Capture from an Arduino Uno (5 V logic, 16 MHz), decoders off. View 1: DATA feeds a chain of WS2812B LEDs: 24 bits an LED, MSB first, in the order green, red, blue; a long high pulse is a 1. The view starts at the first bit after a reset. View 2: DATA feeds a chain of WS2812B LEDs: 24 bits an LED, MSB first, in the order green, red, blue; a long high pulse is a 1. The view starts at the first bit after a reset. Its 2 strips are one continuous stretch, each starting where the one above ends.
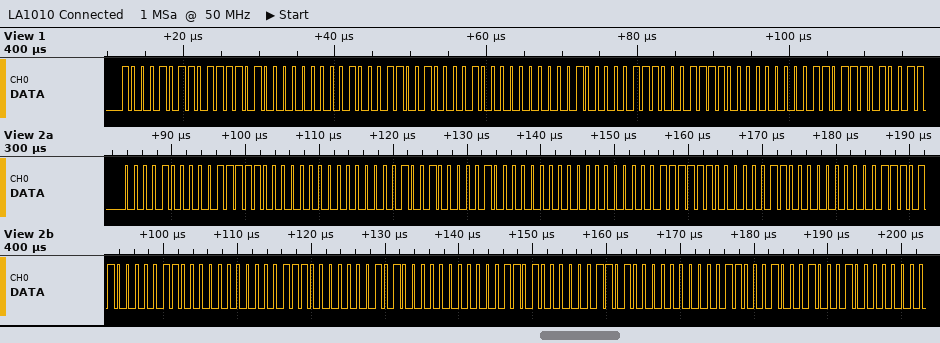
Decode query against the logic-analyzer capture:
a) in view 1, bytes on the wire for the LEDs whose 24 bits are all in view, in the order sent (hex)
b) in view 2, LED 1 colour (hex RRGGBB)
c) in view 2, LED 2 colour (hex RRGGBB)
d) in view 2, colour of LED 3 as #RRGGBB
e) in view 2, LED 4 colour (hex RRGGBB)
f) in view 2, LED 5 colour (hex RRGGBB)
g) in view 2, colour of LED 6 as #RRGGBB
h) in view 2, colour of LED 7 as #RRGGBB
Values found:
8B 7A 00 8C 84 00 83 8F 00
#3E0800
#410200
#3F0003
#3B0006
#38000A
#34000D
#310011
